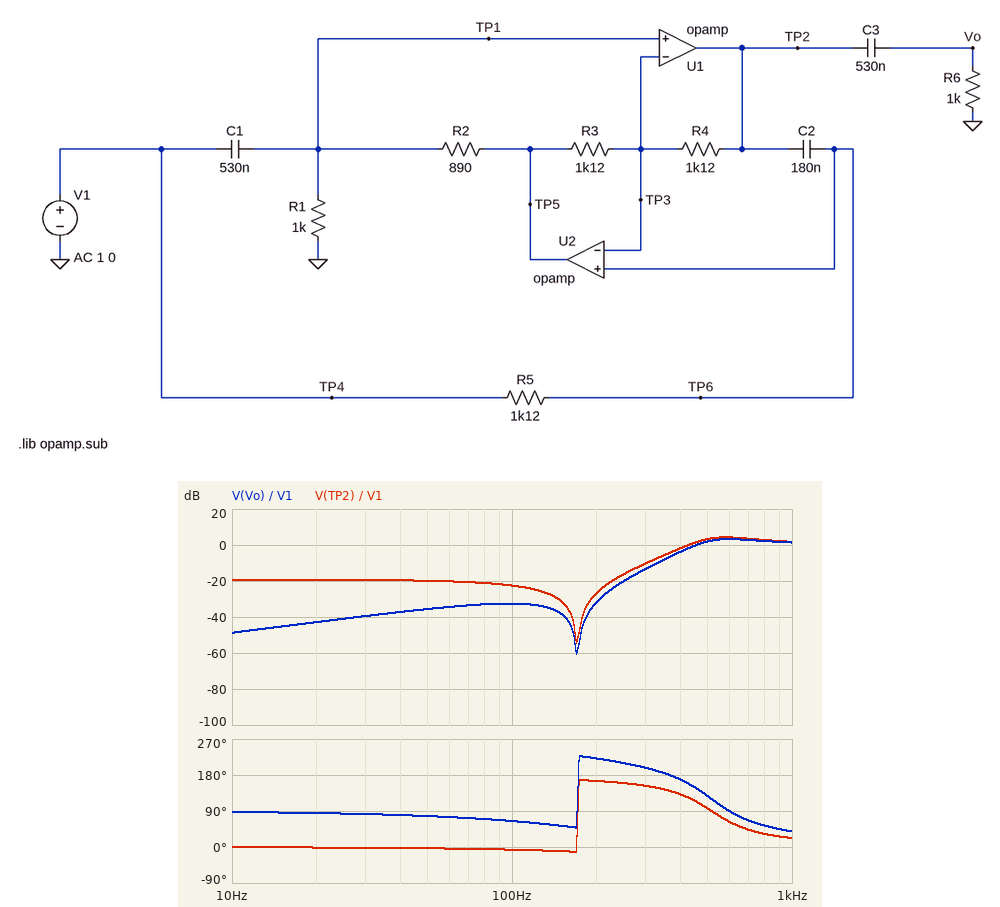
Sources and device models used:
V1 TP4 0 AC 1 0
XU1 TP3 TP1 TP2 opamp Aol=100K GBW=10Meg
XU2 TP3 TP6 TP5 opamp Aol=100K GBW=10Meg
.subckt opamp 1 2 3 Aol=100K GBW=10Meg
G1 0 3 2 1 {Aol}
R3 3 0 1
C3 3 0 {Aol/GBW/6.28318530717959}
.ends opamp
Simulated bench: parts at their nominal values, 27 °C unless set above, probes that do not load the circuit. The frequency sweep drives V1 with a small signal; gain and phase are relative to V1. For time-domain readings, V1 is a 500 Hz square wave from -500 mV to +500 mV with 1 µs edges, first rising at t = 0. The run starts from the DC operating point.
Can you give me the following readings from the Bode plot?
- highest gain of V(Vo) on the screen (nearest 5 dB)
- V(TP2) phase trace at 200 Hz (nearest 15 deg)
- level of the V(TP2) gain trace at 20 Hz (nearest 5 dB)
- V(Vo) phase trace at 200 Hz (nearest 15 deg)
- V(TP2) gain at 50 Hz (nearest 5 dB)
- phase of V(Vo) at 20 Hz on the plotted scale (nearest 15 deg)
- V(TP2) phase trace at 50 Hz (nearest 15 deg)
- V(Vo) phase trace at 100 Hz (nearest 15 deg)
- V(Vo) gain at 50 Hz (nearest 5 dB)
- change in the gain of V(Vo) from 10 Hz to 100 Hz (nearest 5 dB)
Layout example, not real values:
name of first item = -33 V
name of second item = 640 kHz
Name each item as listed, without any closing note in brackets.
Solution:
highest gain of V(Vo) on the screen = 5 dB
V(TP2) phase trace at 200 Hz = 165 deg
level of the V(TP2) gain trace at 20 Hz = -20 dB
V(Vo) phase trace at 200 Hz = 225 deg
V(TP2) gain at 50 Hz = -20 dB
phase of V(Vo) at 20 Hz on the plotted scale = 90 deg
V(TP2) phase trace at 50 Hz = 0 deg
V(Vo) phase trace at 100 Hz = 60 deg
V(Vo) gain at 50 Hz = -35 dB
change in the gain of V(Vo) from 10 Hz to 100 Hz = 15 dB
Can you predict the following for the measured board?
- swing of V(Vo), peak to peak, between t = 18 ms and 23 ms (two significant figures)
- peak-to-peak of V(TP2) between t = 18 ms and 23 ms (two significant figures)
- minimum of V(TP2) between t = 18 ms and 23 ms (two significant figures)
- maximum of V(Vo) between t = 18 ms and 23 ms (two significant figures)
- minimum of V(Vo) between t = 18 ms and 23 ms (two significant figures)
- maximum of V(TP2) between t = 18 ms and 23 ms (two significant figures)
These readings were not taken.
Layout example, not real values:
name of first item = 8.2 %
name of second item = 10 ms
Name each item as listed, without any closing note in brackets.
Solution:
swing of V(Vo), peak to peak, between t = 18 ms and 23 ms = 2.7 V
peak-to-peak of V(TP2) between t = 18 ms and 23 ms = 3.1 V
minimum of V(TP2) between t = 18 ms and 23 ms = -1.5 V
maximum of V(Vo) between t = 18 ms and 23 ms = 1.3 V
minimum of V(Vo) between t = 18 ms and 23 ms = -1.3 V
maximum of V(TP2) between t = 18 ms and 23 ms = 1.5 V
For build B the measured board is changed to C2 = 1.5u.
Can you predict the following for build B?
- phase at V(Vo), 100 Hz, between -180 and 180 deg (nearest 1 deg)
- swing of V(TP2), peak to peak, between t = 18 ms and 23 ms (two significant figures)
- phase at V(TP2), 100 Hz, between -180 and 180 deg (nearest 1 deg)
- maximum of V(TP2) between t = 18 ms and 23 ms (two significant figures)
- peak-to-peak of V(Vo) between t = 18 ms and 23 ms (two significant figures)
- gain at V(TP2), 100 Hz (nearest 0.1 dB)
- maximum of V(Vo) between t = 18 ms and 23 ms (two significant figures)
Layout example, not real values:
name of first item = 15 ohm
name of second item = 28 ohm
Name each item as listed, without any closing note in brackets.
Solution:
phase at V(Vo), 100 Hz, between -180 and 180 deg = -162 deg
swing of V(TP2), peak to peak, between t = 18 ms and 23 ms = 1.9 V
phase at V(TP2), 100 Hz, between -180 and 180 deg = 126 deg
maximum of V(TP2) between t = 18 ms and 23 ms = 930 mV
peak-to-peak of V(Vo) between t = 18 ms and 23 ms = 2.3 V
gain at V(TP2), 100 Hz = -15.2 dB
maximum of V(Vo) between t = 18 ms and 23 ms = 1.1 V
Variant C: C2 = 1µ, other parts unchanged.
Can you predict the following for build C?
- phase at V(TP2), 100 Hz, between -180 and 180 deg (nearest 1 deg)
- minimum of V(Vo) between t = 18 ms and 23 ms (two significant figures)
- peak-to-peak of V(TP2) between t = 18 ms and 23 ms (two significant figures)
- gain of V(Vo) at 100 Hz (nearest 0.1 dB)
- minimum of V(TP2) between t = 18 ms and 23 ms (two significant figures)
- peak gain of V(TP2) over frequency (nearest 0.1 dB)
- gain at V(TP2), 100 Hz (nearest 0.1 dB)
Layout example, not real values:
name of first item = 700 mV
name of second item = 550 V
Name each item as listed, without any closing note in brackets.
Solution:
phase at V(TP2), 100 Hz, between -180 and 180 deg = 142 deg
minimum of V(Vo) between t = 18 ms and 23 ms = -1.2 V
peak-to-peak of V(TP2) between t = 18 ms and 23 ms = 1.9 V
gain of V(Vo) at 100 Hz = -30.2 dB
minimum of V(TP2) between t = 18 ms and 23 ms = -970 mV
peak gain of V(TP2) over frequency = 0 dB
gain at V(TP2), 100 Hz = -20.2 dB
